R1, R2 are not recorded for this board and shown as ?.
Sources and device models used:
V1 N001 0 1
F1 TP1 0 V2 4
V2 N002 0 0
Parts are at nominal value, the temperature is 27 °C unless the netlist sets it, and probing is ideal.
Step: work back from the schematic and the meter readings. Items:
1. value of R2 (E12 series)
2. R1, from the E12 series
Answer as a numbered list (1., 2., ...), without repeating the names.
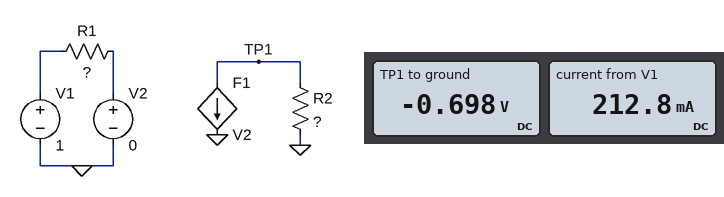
1. 0.82 Ω
2. 4.7 Ω
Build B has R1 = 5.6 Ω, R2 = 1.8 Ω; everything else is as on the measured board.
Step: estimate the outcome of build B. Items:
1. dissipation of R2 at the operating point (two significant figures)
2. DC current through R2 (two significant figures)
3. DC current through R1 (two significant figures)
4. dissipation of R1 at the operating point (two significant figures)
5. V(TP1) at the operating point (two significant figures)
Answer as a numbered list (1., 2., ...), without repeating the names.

1. 920 mW
2. 710 mA
3. 180 mA
4. 180 mW
5. -1.3 V
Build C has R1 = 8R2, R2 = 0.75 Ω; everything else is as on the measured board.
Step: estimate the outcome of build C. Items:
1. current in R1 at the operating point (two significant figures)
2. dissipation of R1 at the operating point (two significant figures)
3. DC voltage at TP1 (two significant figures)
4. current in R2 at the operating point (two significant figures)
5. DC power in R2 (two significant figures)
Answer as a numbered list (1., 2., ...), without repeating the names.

1. 120 mA
2. 120 mW
3. -370 mV
4. 490 mA
5. 180 mW
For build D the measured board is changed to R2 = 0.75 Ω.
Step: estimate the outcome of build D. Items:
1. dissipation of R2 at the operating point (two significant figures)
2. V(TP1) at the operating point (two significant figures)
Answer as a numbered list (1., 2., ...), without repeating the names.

1. 540 mW
2. -640 mV
